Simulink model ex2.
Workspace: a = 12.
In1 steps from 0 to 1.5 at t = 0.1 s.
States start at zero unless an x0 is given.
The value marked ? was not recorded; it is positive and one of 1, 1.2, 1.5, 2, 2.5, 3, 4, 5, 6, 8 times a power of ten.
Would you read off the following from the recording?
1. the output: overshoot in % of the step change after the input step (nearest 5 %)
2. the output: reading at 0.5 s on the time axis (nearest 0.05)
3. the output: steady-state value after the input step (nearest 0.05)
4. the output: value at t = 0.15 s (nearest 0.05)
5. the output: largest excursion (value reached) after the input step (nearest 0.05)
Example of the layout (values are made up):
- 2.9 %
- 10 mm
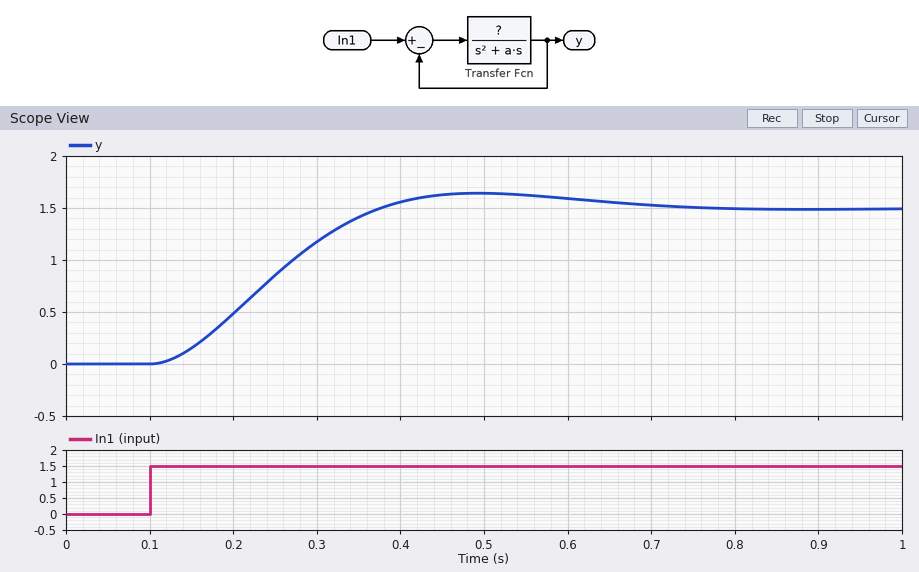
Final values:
- 10 %
- 1.65
- 1.50
- 0.15
- 1.65
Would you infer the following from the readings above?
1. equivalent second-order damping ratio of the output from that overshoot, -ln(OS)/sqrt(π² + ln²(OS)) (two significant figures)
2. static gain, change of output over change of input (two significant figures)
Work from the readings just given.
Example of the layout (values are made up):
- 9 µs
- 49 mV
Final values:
- 0.59
- 1.0
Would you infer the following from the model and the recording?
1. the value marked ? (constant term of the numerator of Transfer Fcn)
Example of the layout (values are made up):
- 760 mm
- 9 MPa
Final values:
- 100
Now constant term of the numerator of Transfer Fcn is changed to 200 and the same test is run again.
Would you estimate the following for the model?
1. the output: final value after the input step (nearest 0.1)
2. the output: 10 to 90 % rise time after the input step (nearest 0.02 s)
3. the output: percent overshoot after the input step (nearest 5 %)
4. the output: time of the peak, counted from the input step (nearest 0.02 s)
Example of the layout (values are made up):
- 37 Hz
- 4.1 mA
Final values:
- 1.5
- 0.10 s
- 25 %
- 0.24 s
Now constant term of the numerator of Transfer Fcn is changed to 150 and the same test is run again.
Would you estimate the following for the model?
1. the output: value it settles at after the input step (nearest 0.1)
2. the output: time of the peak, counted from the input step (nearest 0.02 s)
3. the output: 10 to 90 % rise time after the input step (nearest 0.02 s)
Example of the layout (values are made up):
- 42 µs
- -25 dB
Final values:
- 1.5
- 0.30 s
- 0.14 s
